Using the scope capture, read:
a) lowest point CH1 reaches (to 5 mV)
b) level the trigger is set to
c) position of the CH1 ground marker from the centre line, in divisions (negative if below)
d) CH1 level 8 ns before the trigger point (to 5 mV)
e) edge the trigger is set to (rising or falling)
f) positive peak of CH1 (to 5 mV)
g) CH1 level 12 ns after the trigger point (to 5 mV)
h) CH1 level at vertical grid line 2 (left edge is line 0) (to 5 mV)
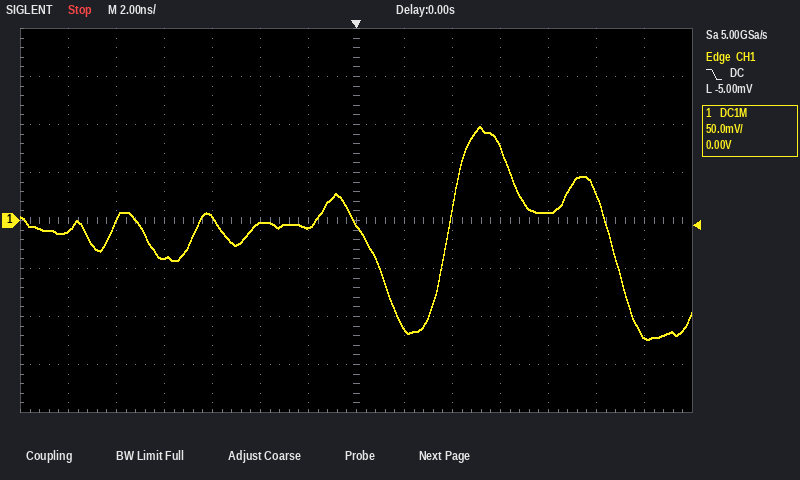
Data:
-125 mV
-5.00 mV
0.0 div
-40 mV
falling
100 mV
-120 mV
0 mV
